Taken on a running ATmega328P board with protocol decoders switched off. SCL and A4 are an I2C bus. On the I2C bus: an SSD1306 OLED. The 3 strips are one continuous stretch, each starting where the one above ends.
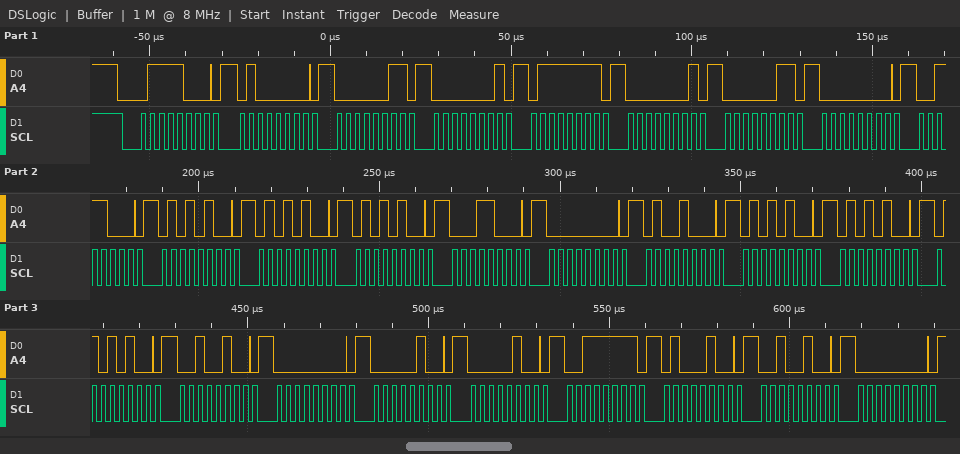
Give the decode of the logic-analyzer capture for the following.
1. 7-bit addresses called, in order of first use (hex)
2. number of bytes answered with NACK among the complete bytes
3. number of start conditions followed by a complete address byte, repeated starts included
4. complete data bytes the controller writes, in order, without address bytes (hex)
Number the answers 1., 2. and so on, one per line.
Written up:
1. 0x3C
2. 0
3. 1
4. 40 03 01 7F 01 03 00 38 54 54 54 18 00 48 54 54 54 24 00 04 04 3F 44 24 00
